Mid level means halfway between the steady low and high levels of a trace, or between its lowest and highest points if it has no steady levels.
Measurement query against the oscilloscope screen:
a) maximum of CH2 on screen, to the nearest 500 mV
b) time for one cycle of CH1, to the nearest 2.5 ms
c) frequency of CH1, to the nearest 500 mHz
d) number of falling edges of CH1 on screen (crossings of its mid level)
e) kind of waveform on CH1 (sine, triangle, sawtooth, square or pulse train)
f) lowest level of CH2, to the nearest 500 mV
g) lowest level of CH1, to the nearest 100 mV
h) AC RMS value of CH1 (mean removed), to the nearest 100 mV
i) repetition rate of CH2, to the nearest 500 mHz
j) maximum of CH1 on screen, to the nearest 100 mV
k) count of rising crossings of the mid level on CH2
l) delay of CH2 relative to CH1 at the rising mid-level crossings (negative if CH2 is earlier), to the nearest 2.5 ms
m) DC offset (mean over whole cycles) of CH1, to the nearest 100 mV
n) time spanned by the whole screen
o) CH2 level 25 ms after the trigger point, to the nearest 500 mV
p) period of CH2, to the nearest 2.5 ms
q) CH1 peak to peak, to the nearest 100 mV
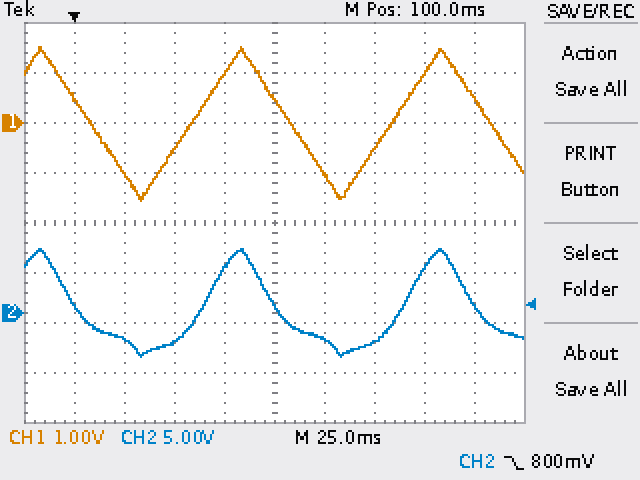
6.5 V
100.0 ms
10.0 Hz
3
triangle
-4.5 V
-1.6 V
900 mV
10.0 Hz
1.5 V
2
+7.5 ms
0.0 V
250 ms
-2.5 V
100.0 ms
3.1 V
